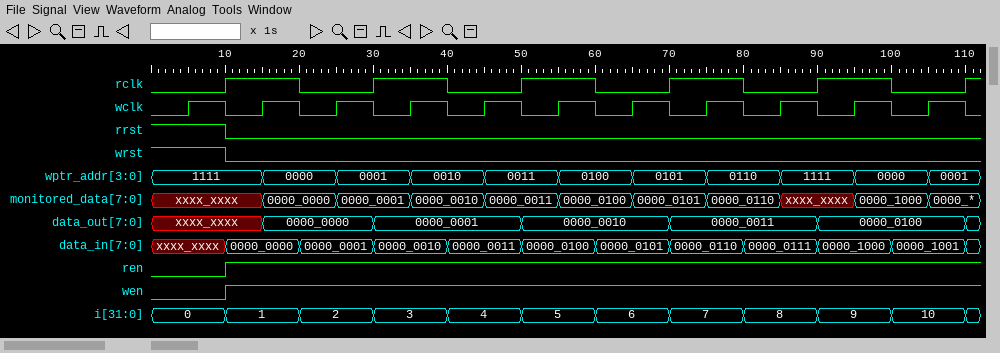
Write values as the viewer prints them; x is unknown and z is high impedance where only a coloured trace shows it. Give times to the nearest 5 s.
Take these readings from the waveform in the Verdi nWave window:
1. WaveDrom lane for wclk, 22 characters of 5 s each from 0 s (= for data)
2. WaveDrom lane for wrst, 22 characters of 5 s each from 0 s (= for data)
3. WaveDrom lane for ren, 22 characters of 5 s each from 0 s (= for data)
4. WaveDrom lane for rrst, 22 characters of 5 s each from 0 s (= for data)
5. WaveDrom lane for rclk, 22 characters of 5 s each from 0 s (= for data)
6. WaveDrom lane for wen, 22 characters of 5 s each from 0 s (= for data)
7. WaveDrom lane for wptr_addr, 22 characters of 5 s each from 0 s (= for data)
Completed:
{name: 'wclk', wave: '0101010101010101010101'}
{name: 'wrst', wave: '1.0...................'}
{name: 'ren', wave: '0.1...................'}
{name: 'rrst', wave: '1.0...................'}
{name: 'rclk', wave: '0.1.0.1.0.1.0.1.0.1.0.'}
{name: 'wen', wave: '0.1...................'}
{name: 'wptr_addr', wave: '=..=.=.=.=.=.=.=.=.=.=', data: '1111 0000 0001 0010 0011 0100 0101 0110 1111 0000 0001'}
